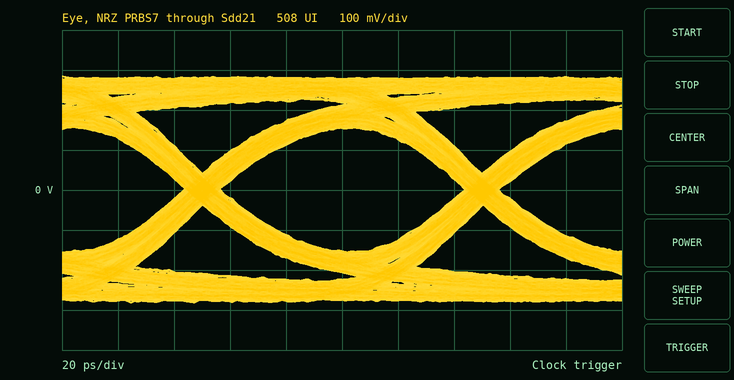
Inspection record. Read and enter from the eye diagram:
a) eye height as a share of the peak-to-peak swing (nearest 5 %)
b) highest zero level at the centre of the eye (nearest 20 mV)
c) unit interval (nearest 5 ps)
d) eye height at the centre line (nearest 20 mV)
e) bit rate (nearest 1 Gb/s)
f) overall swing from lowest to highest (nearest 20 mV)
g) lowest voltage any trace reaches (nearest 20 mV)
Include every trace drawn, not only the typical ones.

55 %
-160 mV
100 ps
300 mV
10 Gb/s
560 mV
-280 mV
